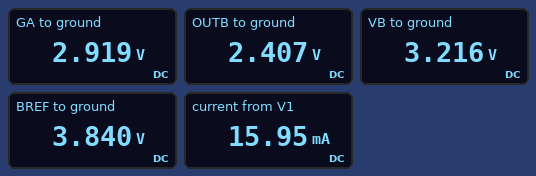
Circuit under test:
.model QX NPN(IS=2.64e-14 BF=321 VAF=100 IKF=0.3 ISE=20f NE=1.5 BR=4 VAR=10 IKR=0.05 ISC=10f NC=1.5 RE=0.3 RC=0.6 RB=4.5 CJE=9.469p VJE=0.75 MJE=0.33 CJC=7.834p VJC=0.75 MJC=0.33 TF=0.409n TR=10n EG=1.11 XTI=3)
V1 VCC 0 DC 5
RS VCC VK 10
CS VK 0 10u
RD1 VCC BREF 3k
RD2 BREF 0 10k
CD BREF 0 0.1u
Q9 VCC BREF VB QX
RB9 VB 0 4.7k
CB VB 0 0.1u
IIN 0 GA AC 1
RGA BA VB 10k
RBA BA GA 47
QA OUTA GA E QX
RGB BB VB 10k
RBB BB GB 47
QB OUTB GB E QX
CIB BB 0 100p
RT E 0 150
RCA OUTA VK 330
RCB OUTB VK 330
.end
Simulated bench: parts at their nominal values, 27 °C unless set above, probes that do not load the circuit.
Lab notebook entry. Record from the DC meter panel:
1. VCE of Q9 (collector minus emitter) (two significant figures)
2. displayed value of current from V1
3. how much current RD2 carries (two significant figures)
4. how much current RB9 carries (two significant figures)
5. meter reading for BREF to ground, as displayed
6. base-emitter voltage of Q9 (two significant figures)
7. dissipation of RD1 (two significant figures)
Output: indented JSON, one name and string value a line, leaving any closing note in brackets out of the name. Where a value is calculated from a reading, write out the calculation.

{
  "VCE of Q9 (collector minus emitter)": "5 V - 3.216 V = 1.8 V",
  "displayed value of current from V1": "15.95 mA",
  "how much current RD2 carries": "(3.84 V) / 10 kΩ = 380 µA",
  "how much current RB9 carries": "(3.216 V) / 4.7 kΩ = 680 µA",
  "meter reading for BREF to ground, as displayed": "3.840 V",
  "base-emitter voltage of Q9": "3.84 V - 3.216 V = 620 mV",
  "dissipation of RD1": "(5 V - 3.84 V)^2 / 3 kΩ = 450 µW"
}
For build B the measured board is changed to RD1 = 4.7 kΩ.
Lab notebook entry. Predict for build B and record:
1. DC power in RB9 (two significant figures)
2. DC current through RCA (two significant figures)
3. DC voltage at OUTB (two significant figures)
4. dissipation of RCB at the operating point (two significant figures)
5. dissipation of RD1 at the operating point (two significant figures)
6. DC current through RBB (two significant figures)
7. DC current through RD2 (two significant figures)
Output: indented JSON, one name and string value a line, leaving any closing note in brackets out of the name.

{
  "DC power in RB9": "1.6 mW",
  "DC current through RCA": "6.2 mA",
  "DC voltage at OUTB": "2.8 V",
  "dissipation of RCB at the operating point": "13 mW",
  "dissipation of RD1 at the operating point": "550 µW",
  "DC current through RBB": "22 µA",
  "DC current through RD2": "340 µA"
}
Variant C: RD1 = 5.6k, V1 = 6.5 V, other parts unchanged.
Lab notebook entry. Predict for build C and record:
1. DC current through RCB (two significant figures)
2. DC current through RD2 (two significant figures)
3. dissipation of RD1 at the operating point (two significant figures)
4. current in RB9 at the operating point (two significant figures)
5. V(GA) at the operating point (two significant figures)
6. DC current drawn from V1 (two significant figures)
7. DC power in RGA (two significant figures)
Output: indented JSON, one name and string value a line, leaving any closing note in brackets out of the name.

{
  "DC current through RCB": "8.4 mA",
  "DC current through RD2": "420 µA",
  "dissipation of RD1 at the operating point": "980 µW",
  "current in RB9 at the operating point": "750 µA",
  "V(GA) at the operating point": "3.2 V",
  "DC current drawn from V1": "18 mA",
  "DC power in RGA": "9.0 µW"
}
